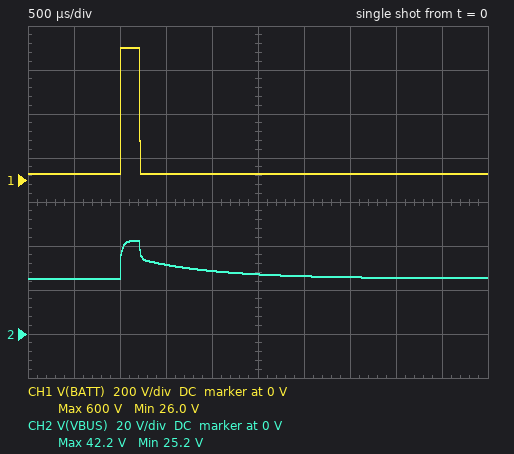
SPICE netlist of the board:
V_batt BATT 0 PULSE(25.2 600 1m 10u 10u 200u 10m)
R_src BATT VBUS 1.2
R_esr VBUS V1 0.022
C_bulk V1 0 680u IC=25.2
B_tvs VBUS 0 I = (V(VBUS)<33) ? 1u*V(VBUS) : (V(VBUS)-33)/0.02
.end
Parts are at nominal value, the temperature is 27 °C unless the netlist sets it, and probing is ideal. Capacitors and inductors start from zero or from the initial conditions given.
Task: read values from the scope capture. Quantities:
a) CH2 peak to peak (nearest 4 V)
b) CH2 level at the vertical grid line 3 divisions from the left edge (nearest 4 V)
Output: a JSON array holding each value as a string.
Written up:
["16 V", "32 V"]
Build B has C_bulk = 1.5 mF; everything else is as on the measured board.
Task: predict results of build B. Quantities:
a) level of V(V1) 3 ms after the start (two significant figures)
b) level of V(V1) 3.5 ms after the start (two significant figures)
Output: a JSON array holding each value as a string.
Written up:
["29 V", "28 V"]
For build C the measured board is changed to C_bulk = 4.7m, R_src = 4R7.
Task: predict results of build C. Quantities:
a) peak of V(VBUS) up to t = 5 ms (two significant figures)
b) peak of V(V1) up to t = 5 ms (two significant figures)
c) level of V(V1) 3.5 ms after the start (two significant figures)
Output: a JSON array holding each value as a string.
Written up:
["33 V", "31 V", "30 V"]
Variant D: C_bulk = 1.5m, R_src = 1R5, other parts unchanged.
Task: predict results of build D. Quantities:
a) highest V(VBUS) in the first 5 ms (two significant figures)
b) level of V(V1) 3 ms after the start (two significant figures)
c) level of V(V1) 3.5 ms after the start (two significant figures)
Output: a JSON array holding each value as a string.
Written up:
["40 V", "29 V", "28 V"]
